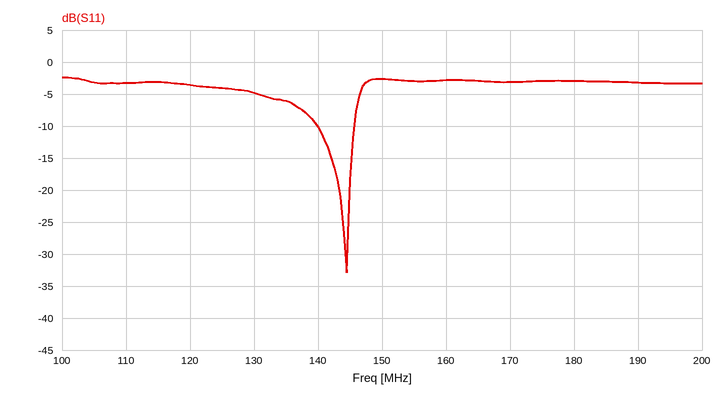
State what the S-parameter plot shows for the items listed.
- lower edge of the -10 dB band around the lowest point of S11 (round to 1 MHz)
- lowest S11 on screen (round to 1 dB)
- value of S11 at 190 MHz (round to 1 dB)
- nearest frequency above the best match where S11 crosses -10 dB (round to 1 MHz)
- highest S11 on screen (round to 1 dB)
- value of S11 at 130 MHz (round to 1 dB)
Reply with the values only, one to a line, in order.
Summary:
140 MHz
-33 dB
-3 dB
146 MHz
-2 dB
-5 dB
